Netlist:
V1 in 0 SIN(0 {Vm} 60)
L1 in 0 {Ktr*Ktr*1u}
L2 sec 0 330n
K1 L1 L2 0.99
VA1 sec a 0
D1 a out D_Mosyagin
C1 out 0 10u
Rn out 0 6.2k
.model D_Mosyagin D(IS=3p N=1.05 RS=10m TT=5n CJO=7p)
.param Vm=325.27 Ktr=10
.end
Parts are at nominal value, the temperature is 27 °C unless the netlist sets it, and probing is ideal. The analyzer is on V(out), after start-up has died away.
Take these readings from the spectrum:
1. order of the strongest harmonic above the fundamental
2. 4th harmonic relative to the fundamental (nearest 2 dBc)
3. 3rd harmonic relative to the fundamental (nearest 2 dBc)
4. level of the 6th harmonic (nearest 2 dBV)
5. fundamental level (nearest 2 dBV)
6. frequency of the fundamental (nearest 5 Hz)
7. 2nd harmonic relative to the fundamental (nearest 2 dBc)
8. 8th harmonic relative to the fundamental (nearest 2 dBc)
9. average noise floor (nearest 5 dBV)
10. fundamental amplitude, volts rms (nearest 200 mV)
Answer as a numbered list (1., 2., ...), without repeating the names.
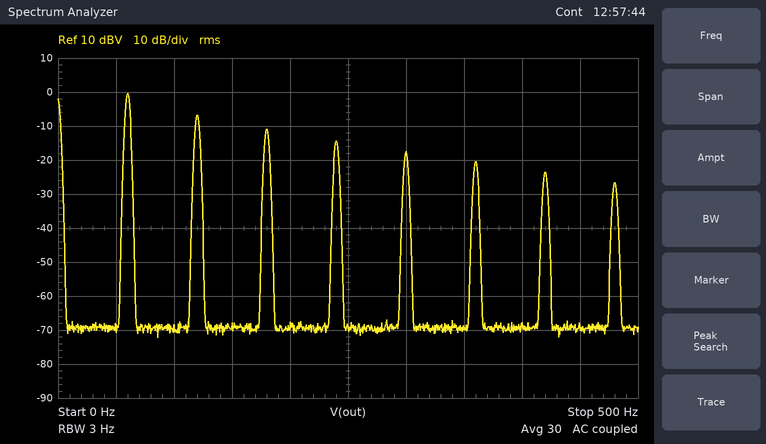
1. 2
2. -14 dBc
3. -10 dBc
4. -20 dBV
5. 0 dBV
6. 60 Hz
7. -6 dBc
8. -26 dBc
9. -70 dBV
10. 1.0 V
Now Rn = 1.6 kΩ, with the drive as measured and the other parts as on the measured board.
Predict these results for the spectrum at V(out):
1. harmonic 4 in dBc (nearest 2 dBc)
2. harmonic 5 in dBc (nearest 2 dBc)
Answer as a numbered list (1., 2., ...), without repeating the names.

1. -18 dBc
2. -24 dBc
